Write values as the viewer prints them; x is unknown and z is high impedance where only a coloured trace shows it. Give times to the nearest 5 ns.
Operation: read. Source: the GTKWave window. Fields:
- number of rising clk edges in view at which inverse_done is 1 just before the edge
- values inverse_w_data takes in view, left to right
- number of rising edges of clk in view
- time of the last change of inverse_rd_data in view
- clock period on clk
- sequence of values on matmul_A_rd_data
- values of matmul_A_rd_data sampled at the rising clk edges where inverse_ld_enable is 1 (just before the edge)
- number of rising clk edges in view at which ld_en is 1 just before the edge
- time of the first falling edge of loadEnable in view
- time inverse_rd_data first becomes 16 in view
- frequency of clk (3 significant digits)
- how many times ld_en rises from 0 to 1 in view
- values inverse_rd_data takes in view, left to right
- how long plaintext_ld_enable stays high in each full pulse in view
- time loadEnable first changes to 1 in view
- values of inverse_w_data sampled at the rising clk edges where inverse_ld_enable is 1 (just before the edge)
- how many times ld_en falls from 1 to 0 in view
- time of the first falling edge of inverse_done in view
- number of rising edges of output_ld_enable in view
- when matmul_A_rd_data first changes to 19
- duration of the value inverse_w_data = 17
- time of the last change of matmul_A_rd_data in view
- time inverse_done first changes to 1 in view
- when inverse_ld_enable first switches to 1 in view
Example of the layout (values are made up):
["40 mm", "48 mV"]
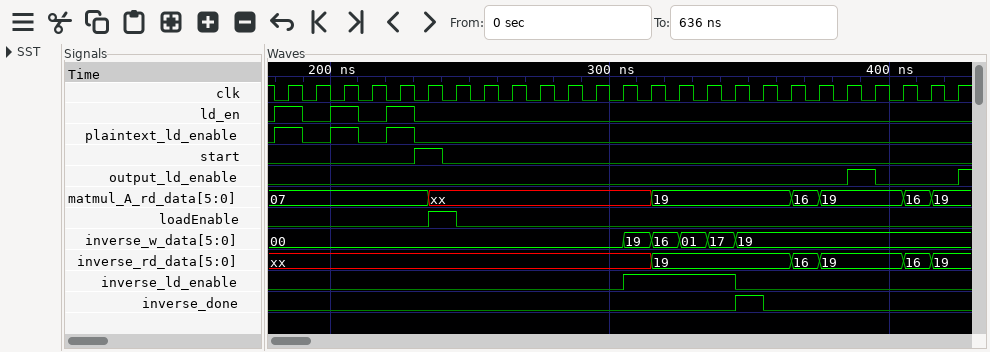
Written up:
["1", "00, 19, 16, 01, 17, 19", "25", "415 ns", "10 ns", "07, xx, 19, 16, 19, 16, 19", "xx, 19, 19, 19", "3", "245 ns", "365 ns", "100 MHz", "3", "xx, 19, 16, 19, 16, 19", "10 ns, 10 ns, 10 ns", "235 ns", "19, 16, 01, 17", "3", "355 ns", "2", "315 ns", "10 ns", "415 ns", "345 ns", "305 ns"]
